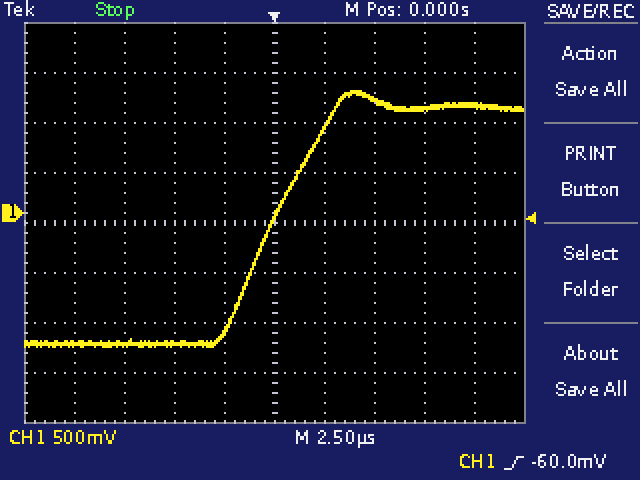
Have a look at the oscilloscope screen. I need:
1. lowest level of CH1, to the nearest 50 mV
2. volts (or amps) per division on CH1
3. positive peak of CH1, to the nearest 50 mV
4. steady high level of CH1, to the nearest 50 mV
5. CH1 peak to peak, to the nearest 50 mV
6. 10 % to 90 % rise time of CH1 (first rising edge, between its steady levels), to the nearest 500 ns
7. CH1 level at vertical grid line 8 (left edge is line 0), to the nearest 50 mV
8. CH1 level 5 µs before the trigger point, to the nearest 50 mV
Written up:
-1.35 V
500 mV
1.20 V
1.05 V
2.55 V
4.5 µs
1.05 V
-1.30 V
